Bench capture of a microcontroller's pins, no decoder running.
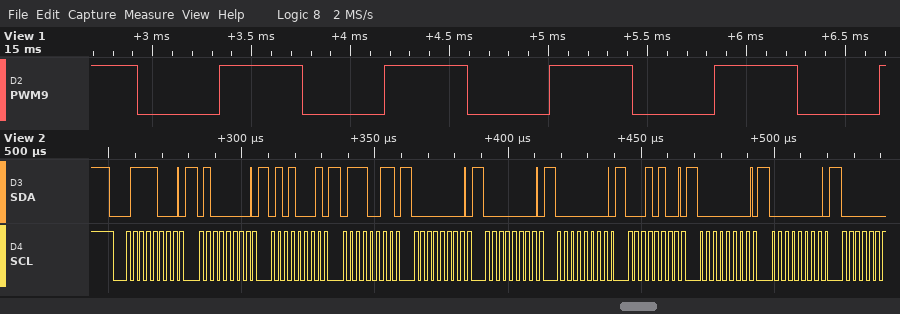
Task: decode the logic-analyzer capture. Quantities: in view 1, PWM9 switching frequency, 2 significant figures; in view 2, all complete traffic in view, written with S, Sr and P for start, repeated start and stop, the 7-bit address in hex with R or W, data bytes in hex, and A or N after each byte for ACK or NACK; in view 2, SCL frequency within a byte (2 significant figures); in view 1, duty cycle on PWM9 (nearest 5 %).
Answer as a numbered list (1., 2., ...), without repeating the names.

1. 1.2 kHz
2. S 3CW A 40 A 51 A 73 A 00 A 00 A 00 A 14 A 00 A 00 A
3. 400 kHz
4. 50 %
